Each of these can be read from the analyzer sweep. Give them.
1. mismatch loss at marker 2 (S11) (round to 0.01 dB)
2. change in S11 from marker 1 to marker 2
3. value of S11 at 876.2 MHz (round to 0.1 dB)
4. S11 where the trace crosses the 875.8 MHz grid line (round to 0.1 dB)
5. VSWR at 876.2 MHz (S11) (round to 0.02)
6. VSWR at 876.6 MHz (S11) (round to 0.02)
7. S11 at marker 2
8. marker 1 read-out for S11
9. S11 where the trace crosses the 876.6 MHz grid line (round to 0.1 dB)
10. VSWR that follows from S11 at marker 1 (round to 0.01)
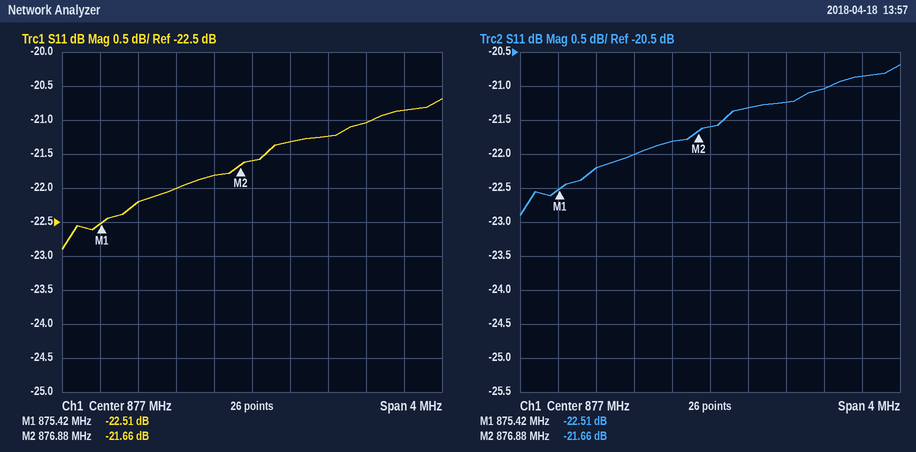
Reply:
0.03 dB
0.85 dB
-22.0 dB
-22.2 dB
1.18
1.18
-21.66 dB
-22.51 dB
-21.8 dB
1.16
